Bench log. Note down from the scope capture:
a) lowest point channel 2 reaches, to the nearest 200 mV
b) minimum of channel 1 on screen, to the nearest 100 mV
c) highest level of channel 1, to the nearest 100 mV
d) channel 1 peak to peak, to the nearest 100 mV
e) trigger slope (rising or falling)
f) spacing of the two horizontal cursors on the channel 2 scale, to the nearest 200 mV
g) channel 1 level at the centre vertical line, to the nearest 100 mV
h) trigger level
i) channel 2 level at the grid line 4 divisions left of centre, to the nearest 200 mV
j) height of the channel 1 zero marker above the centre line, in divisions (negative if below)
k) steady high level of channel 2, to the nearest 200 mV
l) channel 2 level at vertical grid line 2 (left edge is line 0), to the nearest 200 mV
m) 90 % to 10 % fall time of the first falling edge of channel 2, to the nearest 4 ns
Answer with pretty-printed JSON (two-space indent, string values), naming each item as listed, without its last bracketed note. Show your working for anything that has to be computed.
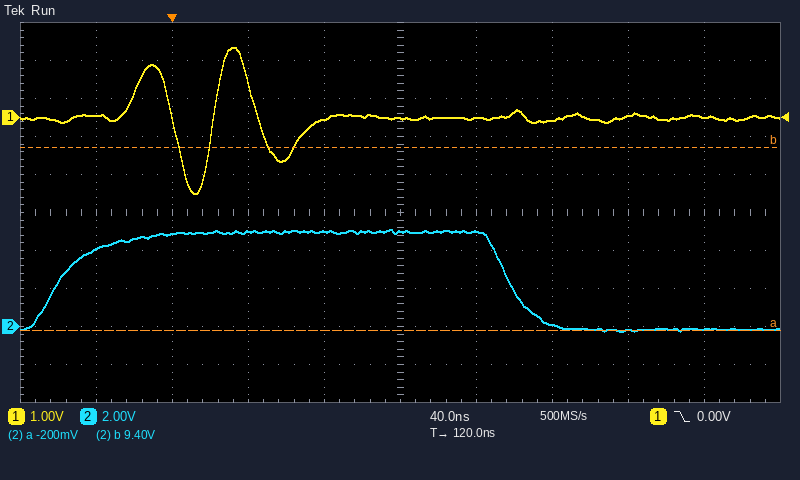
{
  "lowest point channel 2 reaches, to the nearest 200 mV": "-200 mV",
  "minimum of channel 1 on screen, to the nearest 100 mV": "-2.0 V",
  "highest level of channel 1, to the nearest 100 mV": "1.8 V",
  "channel 1 peak to peak, to the nearest 100 mV": "1.8 V − (-2.0 V) = 3.8 V",
  "trigger slope": "falling",
  "spacing of the two horizontal cursors on the channel 2 scale, to the nearest 200 mV": "9.6 V",
  "channel 1 level at the centre vertical line, to the nearest 100 mV": "0.0 V",
  "trigger level": "0.00 V",
  "channel 2 level at the grid line 4 divisions left of centre, to the nearest 200 mV": "4.0 V",
  "height of the channel 1 zero marker above the centre line, in divisions": "+2.5 div",
  "steady high level of channel 2, to the nearest 200 mV": "5.0 V",
  "channel 2 level at vertical grid line 2 (left edge is line 0), to the nearest 200 mV": "4.8 V",
  "90 % to 10 % fall time of the first falling edge of channel 2, to the nearest 4 ns": "28 ns"
}
